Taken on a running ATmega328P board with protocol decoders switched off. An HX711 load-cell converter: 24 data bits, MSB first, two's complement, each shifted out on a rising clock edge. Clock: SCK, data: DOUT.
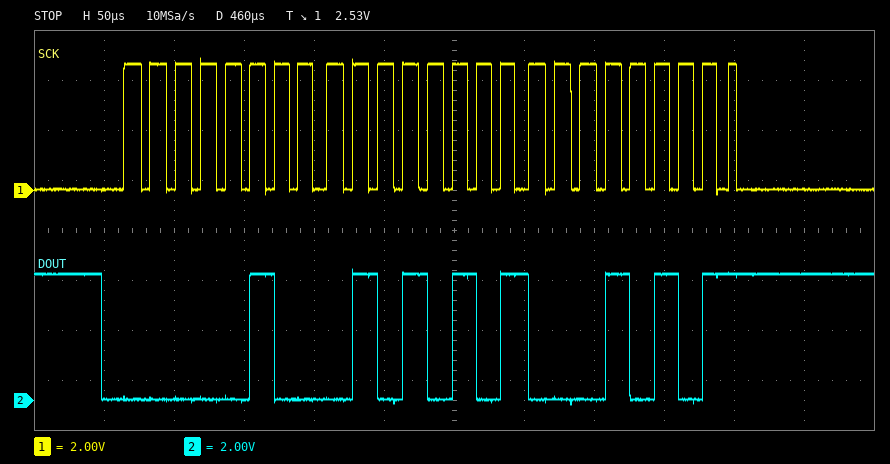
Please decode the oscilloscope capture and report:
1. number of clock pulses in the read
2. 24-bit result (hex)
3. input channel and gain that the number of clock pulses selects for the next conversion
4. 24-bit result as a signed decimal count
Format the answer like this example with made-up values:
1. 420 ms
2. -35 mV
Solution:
1. 25
2. 0x045515
3. channel A, gain 128
4. 283925
